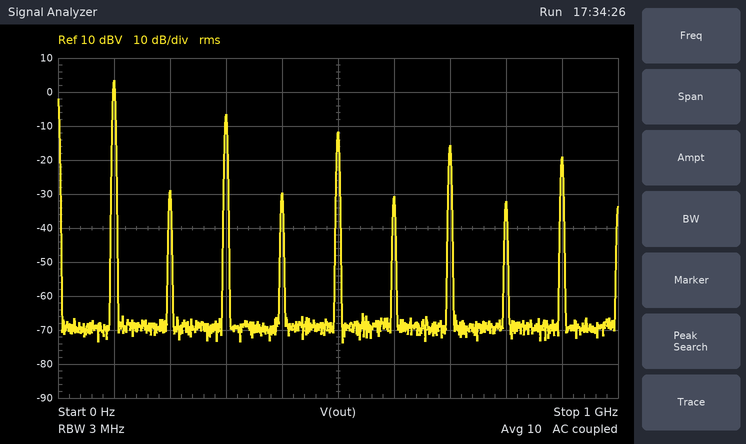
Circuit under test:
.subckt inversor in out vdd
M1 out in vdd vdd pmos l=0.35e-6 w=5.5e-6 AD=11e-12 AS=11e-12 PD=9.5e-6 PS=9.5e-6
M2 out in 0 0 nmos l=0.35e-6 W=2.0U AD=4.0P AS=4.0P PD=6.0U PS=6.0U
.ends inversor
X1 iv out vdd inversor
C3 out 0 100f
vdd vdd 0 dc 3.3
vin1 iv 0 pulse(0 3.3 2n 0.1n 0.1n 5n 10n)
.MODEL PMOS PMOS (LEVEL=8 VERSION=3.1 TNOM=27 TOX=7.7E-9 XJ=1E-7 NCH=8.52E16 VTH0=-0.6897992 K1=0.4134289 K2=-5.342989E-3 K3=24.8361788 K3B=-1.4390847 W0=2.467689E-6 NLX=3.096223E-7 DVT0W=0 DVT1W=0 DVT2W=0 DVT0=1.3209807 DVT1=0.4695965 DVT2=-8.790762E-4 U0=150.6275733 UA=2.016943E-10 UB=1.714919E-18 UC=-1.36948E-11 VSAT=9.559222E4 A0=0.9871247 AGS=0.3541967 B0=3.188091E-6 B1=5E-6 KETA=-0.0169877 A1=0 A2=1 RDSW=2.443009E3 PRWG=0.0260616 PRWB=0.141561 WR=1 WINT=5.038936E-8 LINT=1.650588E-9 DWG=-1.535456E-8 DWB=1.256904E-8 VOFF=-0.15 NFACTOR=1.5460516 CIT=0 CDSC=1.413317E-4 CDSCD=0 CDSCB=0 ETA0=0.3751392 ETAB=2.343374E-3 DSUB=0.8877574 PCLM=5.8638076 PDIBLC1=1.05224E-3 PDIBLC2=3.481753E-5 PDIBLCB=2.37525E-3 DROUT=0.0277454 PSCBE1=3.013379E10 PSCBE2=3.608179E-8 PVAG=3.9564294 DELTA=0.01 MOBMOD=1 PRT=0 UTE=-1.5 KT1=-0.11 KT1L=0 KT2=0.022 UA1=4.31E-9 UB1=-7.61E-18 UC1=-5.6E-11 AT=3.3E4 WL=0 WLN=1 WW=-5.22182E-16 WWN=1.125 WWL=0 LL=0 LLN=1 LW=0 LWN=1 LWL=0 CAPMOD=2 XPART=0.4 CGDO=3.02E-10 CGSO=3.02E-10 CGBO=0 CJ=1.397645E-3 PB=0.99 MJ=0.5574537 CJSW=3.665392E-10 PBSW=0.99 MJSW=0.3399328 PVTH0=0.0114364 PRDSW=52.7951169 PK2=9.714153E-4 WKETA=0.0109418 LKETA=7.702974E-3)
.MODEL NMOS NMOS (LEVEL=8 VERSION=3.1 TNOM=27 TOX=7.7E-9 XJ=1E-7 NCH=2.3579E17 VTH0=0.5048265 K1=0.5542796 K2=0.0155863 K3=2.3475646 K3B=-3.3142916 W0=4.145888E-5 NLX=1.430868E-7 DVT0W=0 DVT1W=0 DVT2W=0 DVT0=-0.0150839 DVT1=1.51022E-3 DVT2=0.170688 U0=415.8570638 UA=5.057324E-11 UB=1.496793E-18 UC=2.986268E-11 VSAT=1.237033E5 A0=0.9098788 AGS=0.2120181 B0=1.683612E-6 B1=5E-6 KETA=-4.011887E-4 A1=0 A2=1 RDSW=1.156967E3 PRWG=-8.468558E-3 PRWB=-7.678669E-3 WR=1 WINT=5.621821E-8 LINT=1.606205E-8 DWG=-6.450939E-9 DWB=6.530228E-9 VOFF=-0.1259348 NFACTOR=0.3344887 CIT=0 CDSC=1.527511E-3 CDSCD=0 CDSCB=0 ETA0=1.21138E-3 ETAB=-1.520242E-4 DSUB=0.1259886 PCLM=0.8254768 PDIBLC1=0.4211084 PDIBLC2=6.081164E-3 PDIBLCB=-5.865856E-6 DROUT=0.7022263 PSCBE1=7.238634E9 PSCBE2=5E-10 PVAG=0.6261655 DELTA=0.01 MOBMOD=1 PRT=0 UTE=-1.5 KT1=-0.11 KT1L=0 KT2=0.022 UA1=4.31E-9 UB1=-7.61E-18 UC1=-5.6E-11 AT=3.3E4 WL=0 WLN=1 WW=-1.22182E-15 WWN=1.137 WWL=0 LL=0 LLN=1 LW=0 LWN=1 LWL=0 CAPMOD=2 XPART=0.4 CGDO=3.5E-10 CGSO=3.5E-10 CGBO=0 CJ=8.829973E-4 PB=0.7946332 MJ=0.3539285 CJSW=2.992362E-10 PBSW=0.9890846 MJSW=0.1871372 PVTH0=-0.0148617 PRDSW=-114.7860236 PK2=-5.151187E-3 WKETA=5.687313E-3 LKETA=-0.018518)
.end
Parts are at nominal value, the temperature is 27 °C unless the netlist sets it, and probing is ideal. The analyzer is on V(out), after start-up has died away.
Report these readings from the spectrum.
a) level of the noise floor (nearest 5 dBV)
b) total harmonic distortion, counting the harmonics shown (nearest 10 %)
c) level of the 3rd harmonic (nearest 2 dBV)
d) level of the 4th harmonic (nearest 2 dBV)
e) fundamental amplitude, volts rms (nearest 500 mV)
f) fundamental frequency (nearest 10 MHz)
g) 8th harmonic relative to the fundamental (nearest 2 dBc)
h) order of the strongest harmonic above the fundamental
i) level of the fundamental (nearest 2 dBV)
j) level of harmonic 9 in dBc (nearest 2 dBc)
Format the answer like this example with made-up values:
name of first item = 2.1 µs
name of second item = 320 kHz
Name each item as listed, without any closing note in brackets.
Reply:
level of the noise floor = -70 dBV
total harmonic distortion, counting the harmonics shown = 40 %
level of the 3rd harmonic = -6 dBV
level of the 4th harmonic = -30 dBV
fundamental amplitude, volts rms = 1.5 V
fundamental frequency = 100 MHz
8th harmonic relative to the fundamental = -36 dBc
order of the strongest harmonic above the fundamental = 3
level of the fundamental = 4 dBV
level of harmonic 9 in dBc = -22 dBc
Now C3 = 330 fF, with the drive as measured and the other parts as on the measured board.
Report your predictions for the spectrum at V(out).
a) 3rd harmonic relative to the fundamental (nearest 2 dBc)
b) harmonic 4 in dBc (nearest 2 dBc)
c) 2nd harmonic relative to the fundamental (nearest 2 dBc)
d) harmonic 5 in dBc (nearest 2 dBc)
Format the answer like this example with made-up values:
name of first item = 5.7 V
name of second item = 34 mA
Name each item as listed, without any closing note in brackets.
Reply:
3rd harmonic relative to the fundamental = -12 dBc
harmonic 4 in dBc = -44 dBc
2nd harmonic relative to the fundamental = -40 dBc
harmonic 5 in dBc = -20 dBc
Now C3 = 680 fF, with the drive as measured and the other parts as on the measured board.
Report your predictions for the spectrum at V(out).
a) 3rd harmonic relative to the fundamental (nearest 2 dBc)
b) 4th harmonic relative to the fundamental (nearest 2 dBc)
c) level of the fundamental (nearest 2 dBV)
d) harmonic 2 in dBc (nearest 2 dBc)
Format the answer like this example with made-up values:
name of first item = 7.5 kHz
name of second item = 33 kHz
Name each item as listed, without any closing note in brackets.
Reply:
3rd harmonic relative to the fundamental = -18 dBc
4th harmonic relative to the fundamental = -40 dBc
level of the fundamental = 2 dBV
harmonic 2 in dBc = -40 dBc
